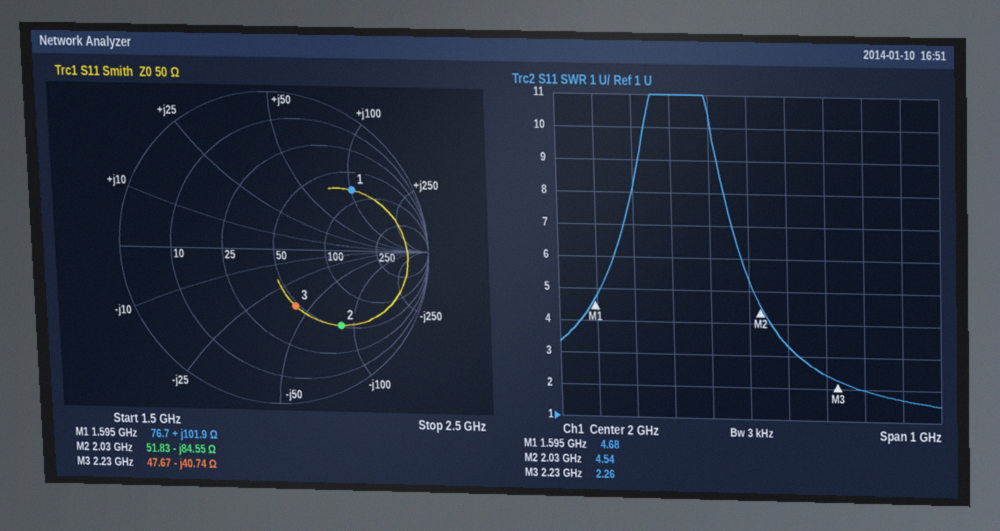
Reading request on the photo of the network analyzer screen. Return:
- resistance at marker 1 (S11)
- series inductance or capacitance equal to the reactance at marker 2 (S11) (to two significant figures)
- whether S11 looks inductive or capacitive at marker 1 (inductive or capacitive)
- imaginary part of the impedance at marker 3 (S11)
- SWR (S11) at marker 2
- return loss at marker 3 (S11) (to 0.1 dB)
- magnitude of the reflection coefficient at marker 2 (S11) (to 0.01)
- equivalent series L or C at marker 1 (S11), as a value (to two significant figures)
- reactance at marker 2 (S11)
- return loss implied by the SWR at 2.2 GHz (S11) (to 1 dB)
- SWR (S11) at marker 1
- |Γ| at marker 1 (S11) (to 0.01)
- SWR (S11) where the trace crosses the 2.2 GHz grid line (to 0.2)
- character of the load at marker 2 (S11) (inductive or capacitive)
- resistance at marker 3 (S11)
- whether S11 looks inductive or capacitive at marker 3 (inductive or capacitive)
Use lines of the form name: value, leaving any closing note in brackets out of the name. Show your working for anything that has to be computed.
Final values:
resistance at marker 1: 76.7 Ω
series inductance or capacitance equal to the reactance at marker 2 (S11): C = 1/(2π × 2.03 GHz × 84.55 Ω) ≈ 927 fF, so 930 fF to two significant figures
whether S11 looks inductive or capacitive at marker 1: inductive
imaginary part of the impedance at marker 3: -40.74 Ω
SWR (S11) at marker 2: 4.54
return loss at marker 3 (S11): 8.3 dB
magnitude of the reflection coefficient at marker 2 (S11): 0.64
equivalent series L or C at marker 1 (S11), as a value: L = 101.9 Ω/(2π × 1.595 GHz) ≈ 10 nH
reactance at marker 2: -84.55 Ω
return loss implied by the SWR at 2.2 GHz (S11): −20 log10((2.4 − 1)/(2.4 + 1)) ≈ 8 dB
SWR (S11) at marker 1: 4.68
|Γ| at marker 1 (S11): 0.65
SWR (S11) where the trace crosses the 2.2 GHz grid line: 2.4
character of the load at marker 2 (S11): capacitive
resistance at marker 3: 47.67 Ω
whether S11 looks inductive or capacitive at marker 3: capacitive
